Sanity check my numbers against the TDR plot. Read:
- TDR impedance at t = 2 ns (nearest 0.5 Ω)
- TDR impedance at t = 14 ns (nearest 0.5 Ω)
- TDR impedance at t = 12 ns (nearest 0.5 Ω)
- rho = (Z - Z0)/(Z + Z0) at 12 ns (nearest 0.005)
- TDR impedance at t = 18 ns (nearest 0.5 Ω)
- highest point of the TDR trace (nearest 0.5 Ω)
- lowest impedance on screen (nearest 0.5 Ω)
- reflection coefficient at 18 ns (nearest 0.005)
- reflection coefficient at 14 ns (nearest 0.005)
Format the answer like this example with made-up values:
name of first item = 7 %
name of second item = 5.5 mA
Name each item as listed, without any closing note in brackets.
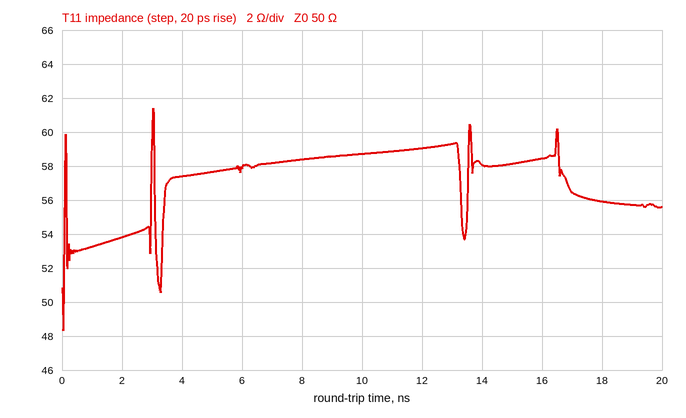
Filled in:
TDR impedance at t = 2 ns = 54.0 Ω
TDR impedance at t = 14 ns = 58.0 Ω
TDR impedance at t = 12 ns = 59.0 Ω
rho = (Z - Z0)/(Z + Z0) at 12 ns = +0.085
TDR impedance at t = 18 ns = 56.0 Ω
highest point of the TDR trace = 61.5 Ω
lowest impedance on screen = 48.5 Ω
reflection coefficient at 18 ns = +0.055
reflection coefficient at 14 ns = +0.075
